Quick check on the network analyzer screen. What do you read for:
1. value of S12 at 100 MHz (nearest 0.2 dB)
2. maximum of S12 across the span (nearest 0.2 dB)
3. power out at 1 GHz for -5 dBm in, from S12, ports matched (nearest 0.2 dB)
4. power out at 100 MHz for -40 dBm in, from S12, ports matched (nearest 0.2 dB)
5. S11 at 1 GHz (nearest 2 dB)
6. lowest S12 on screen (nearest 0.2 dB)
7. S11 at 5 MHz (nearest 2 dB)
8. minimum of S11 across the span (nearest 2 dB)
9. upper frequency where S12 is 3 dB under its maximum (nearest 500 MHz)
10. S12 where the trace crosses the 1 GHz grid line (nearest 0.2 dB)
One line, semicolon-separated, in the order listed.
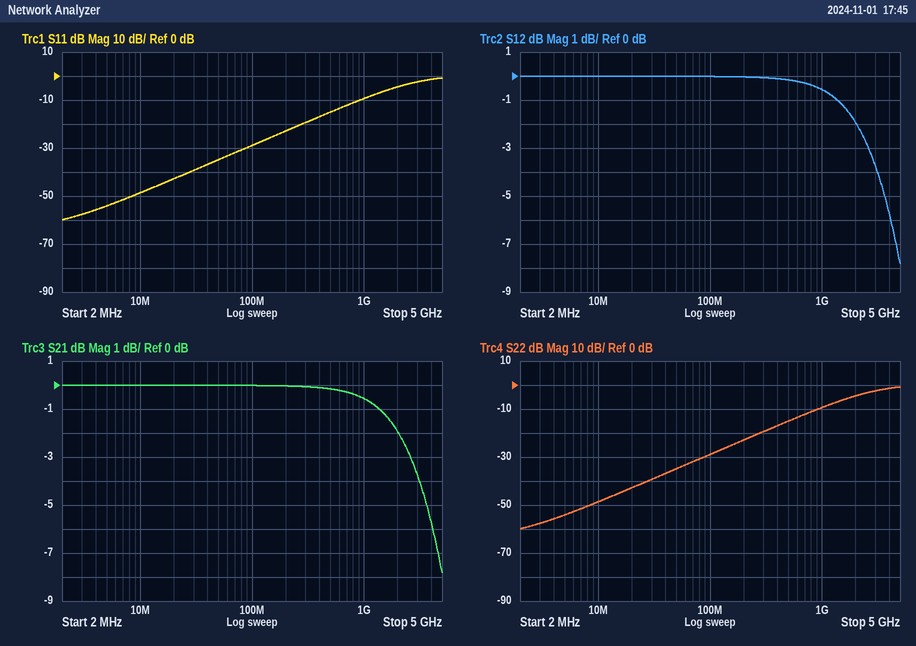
0.0 dB; 0.0 dB; -5.6 dBm; -40.0 dBm; -10 dB; -7.8 dB; -54 dB; -60 dB; 2.5 GHz; -0.6 dB
